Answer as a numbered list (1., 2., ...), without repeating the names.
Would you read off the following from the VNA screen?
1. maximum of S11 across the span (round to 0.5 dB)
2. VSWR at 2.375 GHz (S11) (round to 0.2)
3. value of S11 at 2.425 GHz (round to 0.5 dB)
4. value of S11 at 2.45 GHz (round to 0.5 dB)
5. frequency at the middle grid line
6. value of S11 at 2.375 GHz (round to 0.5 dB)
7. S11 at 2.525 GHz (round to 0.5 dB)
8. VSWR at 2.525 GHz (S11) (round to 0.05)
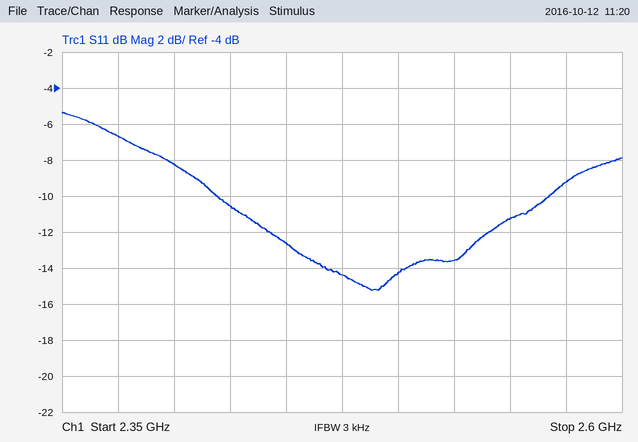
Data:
1. -5.5 dB
2. 2.8
3. -10.5 dB
4. -12.5 dB
5. 2.475 GHz
6. -6.5 dB
7. -13.5 dB
8. 1.55
